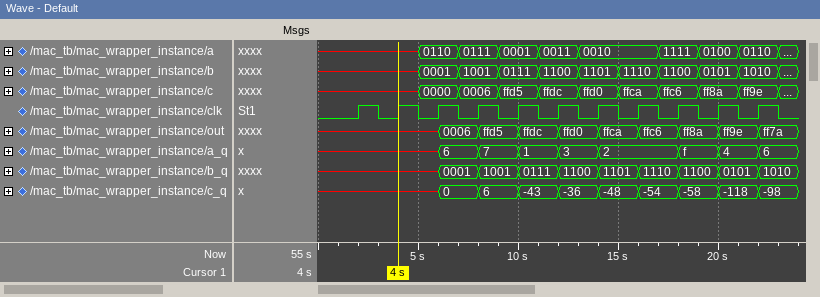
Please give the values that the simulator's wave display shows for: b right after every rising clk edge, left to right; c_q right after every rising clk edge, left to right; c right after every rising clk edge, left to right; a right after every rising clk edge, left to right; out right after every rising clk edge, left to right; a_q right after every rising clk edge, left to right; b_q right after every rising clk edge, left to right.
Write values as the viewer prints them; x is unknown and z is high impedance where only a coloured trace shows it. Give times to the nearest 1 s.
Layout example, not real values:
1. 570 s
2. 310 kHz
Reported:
1. x, x, 0001, 1001, 0111, 1100, 1101, 1110, 1100, 0101, 1010
2. x, x, 0, 6, -43, -36, -48, -54, -58, -118, -98
3. x, x, 0000, 0006, ffd5, ffdc, ffd0, ffca, ffc6, ff8a, ff9e
4. x, x, 0110, 0111, 0001, 0011, 0010, 0010, 1111, 0100, 0110
5. x, x, 0006, ffd5, ffdc, ffd0, ffca, ffc6, ff8a, ff9e, ff7a
6. x, x, 6, 7, 1, 3, 2, 2, f, 4, 6
7. x, x, 0001, 1001, 0111, 1100, 1101, 1110, 1100, 0101, 1010
